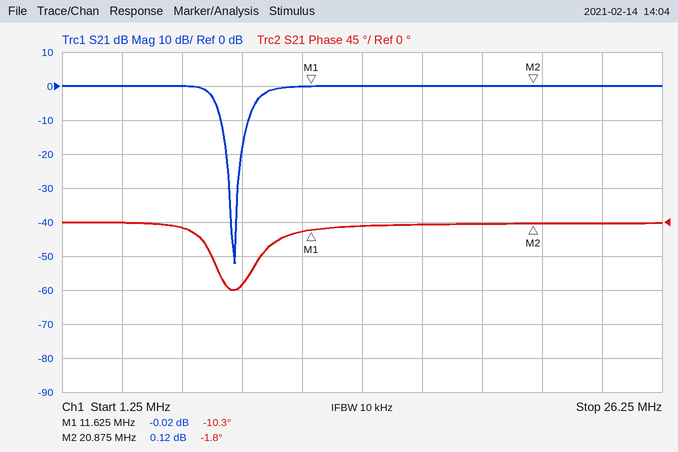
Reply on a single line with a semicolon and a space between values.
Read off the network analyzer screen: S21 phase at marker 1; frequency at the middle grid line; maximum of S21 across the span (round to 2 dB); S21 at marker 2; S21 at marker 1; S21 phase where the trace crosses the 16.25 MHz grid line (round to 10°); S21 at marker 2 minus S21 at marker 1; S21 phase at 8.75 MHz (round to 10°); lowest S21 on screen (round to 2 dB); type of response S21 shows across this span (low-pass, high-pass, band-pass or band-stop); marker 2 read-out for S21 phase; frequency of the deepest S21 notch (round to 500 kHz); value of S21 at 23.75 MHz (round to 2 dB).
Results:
-10.3°; 13.75 MHz; 0 dB; 0.12 dB; -0.02 dB; 0°; 0.14 dB; -80°; -52 dB; band-stop; -1.8°; 8.5 MHz; 0 dB
